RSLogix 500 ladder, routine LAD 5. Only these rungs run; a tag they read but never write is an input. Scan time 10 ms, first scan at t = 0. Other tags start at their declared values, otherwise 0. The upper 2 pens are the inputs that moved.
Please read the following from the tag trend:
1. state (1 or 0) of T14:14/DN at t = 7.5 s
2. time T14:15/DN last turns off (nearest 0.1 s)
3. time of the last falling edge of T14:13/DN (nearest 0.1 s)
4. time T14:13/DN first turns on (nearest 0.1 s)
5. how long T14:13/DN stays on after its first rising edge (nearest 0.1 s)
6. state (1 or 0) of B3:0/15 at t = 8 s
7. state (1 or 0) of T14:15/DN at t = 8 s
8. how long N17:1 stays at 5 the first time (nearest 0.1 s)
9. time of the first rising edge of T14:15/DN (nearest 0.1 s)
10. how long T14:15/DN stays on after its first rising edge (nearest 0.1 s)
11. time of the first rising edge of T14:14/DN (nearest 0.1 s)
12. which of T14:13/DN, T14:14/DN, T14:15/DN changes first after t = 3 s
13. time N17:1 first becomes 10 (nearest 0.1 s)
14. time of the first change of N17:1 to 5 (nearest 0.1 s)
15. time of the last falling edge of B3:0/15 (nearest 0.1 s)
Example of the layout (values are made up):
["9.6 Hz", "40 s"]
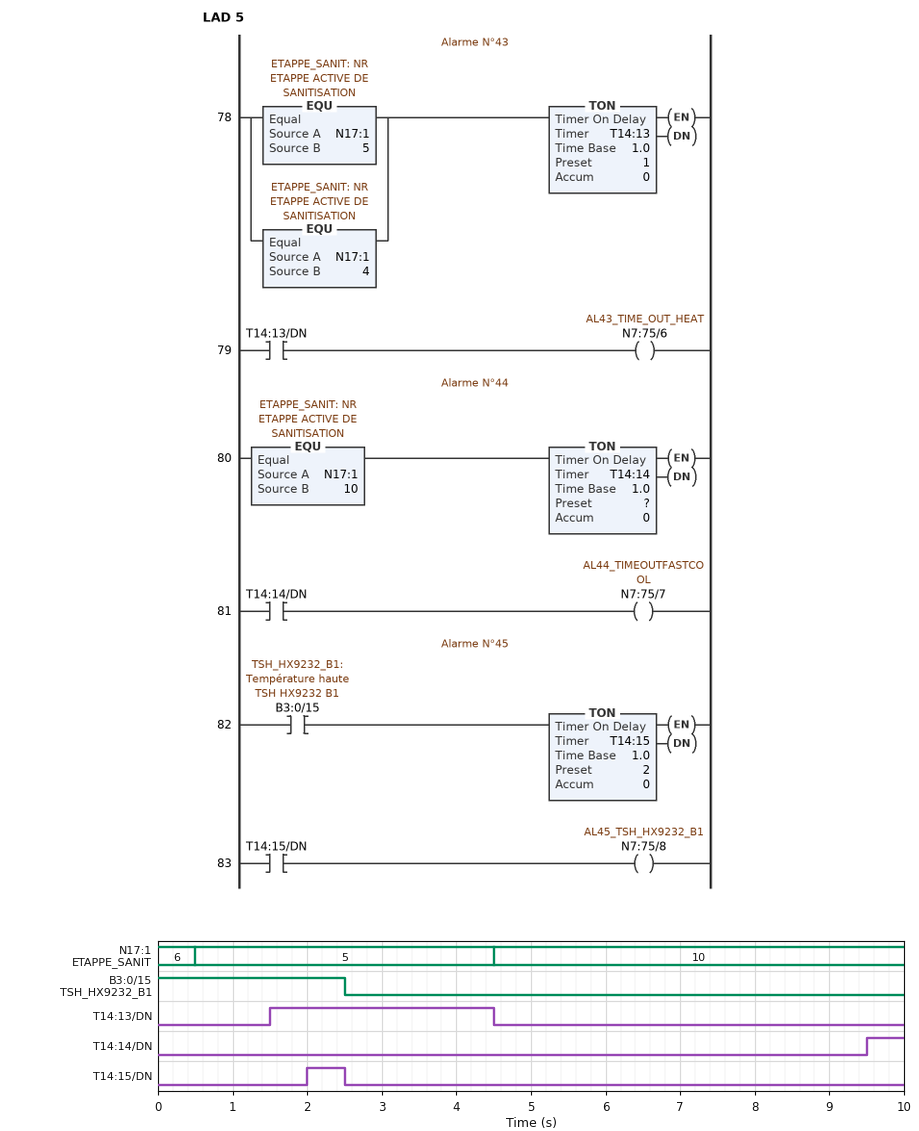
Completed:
["0", "2.5 s", "4.5 s", "1.5 s", "3.0 s", "0", "0", "4.0 s", "2.0 s", "0.5 s", "9.5 s", "T14:13/DN", "4.5 s", "0.5 s", "2.5 s"]
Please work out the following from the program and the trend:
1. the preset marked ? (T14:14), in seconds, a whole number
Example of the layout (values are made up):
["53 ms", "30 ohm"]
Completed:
["5 s"]
